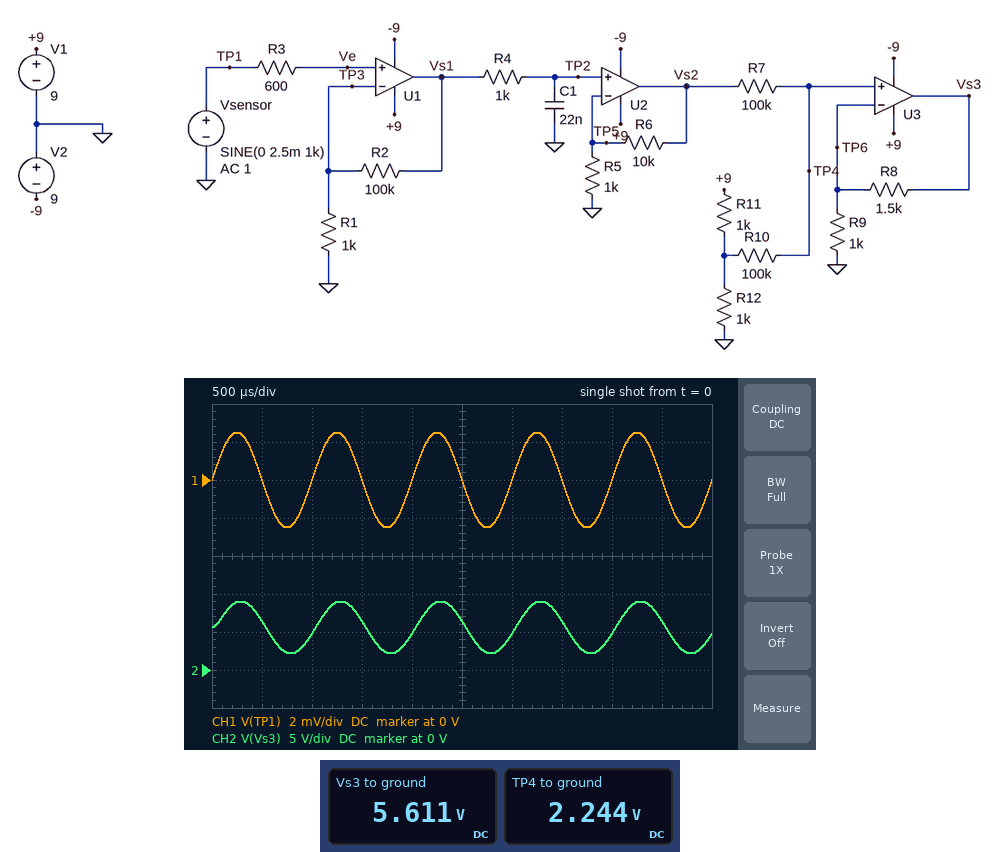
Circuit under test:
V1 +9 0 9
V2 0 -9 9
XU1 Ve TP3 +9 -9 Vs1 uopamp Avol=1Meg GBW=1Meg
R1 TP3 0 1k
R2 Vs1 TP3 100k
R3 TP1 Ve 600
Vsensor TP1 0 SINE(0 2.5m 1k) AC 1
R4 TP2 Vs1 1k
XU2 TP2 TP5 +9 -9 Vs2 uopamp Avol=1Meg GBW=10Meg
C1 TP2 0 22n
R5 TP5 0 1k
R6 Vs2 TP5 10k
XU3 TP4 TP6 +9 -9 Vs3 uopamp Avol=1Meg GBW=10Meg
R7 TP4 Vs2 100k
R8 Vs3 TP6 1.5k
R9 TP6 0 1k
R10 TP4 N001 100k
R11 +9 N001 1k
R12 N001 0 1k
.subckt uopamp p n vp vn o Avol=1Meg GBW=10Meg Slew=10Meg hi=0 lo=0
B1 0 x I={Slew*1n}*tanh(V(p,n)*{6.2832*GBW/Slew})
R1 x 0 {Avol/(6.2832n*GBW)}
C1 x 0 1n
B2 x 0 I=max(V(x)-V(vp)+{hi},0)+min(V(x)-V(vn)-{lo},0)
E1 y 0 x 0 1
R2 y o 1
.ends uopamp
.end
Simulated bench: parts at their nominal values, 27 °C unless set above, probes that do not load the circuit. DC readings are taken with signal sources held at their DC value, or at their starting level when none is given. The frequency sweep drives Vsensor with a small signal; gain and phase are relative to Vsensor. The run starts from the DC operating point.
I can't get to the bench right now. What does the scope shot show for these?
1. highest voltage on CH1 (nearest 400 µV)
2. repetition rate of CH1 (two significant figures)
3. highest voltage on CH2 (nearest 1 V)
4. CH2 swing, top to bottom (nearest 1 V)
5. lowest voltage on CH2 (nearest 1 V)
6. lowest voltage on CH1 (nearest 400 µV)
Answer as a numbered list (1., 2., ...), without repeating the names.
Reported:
1. 2.4 mV
2. 1.0 kHz
3. 9 V
4. 7 V
5. 2 V
6. -2.4 mV
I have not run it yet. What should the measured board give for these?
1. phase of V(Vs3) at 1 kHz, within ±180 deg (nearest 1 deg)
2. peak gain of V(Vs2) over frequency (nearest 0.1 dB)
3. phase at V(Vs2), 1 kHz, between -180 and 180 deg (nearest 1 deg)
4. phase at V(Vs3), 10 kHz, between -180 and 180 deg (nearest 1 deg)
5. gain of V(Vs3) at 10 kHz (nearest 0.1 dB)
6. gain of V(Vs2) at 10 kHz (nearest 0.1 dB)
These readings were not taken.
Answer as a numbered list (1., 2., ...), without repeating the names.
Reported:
1. -14 deg
2. 60.9 dB
3. -14 deg
4. -100 deg
5. 55.2 dB
6. 53.2 dB
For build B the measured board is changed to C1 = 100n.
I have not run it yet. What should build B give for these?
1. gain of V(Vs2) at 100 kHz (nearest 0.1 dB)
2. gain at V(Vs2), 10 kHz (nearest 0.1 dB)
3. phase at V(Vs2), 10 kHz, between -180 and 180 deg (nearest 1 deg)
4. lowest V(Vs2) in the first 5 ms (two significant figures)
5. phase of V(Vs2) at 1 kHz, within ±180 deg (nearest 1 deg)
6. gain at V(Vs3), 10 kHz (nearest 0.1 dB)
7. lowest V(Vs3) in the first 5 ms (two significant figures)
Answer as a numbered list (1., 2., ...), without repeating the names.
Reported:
1. 4.8 dB
2. 41.8 dB
3. -127 deg
4. -2.3 V
5. -38 deg
6. 43.7 dB
7. 2.7 V
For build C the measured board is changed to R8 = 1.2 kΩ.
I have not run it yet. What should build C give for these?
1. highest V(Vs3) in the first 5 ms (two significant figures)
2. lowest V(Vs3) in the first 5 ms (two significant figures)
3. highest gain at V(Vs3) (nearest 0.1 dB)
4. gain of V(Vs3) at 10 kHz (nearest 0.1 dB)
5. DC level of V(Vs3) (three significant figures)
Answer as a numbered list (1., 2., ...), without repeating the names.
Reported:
1. 8.0 V
2. 1.9 V
3. 61.8 dB
4. 54.1 dB
5. 4.94 V
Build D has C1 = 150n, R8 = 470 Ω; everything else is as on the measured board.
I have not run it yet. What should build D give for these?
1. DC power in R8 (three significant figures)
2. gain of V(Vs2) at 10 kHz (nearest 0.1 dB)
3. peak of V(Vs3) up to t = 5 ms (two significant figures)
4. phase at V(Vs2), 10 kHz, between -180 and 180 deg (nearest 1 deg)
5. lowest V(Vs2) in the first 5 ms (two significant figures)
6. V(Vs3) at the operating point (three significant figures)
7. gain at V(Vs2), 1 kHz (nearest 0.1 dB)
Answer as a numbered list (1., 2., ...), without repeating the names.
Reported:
1. 2.37 mW
2. 38.3 dB
3. 4.9 V
4. -130 deg
5. -2.0 V
6. 3.30 V
7. 58.1 dB
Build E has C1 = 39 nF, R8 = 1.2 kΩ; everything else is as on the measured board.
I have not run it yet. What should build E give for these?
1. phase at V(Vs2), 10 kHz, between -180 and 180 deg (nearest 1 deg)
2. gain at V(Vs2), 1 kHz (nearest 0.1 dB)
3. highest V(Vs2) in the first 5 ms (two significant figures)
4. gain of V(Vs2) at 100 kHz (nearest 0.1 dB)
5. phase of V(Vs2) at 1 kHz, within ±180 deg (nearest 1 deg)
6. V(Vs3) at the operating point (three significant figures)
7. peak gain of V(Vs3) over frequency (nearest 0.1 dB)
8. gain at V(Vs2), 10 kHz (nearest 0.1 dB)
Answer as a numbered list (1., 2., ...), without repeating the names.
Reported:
1. -114 deg
2. 60.6 dB
3. 2.7 V
4. 12.9 dB
5. -20 deg
6. 4.94 V
7. 61.8 dB
8. 49.4 dB
